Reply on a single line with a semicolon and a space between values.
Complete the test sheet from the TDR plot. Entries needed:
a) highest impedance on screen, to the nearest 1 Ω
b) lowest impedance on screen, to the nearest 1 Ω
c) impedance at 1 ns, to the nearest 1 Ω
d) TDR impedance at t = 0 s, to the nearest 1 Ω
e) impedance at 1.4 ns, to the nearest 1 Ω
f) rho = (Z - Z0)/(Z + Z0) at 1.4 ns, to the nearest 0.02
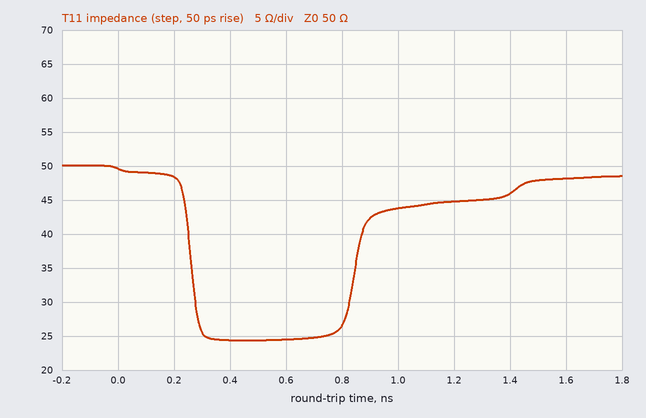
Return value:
50 Ω; 24 Ω; 44 Ω; 50 Ω; 46 Ω; -0.04
